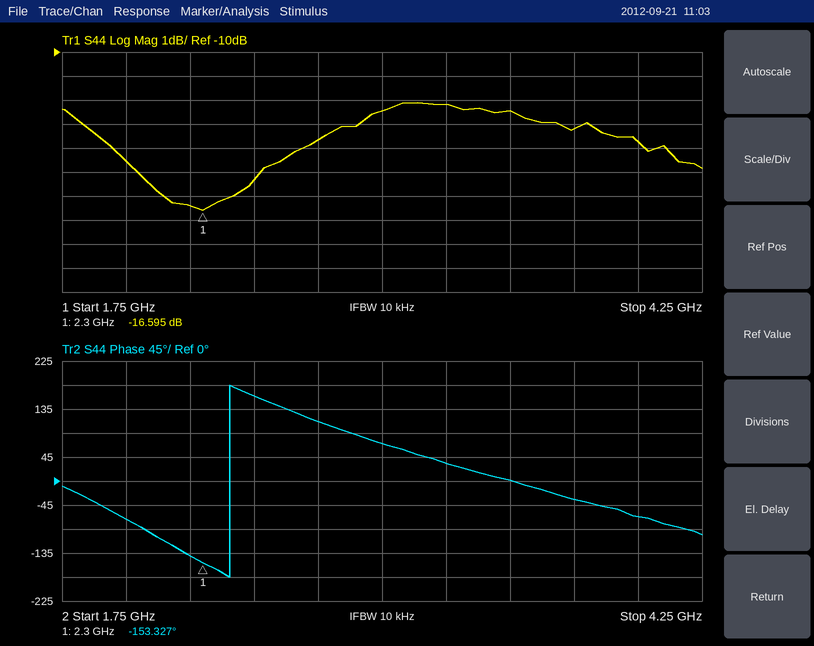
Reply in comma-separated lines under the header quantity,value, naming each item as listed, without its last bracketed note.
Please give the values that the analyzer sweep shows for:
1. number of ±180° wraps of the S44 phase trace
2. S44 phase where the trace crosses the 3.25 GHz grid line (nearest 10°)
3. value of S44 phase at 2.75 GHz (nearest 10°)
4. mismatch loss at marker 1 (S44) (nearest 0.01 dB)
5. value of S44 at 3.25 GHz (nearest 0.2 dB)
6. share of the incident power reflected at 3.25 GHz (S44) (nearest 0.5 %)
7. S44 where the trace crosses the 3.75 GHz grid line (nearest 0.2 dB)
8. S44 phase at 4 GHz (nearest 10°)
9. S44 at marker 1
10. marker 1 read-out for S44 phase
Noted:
quantity,value
number of ±180° wraps of the S44 phase trace,1
S44 phase where the trace crosses the 3.25 GHz grid line,30°
value of S44 phase at 2.75 GHz,110°
mismatch loss at marker 1 (S44),0.10 dB
value of S44 at 3.25 GHz,-12.2 dB
share of the incident power reflected at 3.25 GHz (S44),6.0 %
S44 where the trace crosses the 3.75 GHz grid line,-13.2 dB
S44 phase at 4 GHz,-70°
S44 at marker 1,-16.595 dB
marker 1 read-out for S44 phase,-153.327°
